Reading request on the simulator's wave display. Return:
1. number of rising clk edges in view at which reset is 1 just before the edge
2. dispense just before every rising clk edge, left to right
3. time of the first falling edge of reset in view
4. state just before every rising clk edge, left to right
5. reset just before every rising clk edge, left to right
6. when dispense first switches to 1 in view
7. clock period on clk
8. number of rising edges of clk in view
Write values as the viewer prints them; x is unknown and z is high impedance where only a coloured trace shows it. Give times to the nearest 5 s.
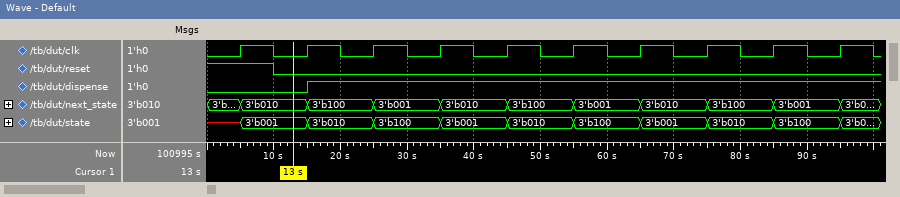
1
0 0 1 1 1 1 1 1 1 1
10 s
x, 3'b001, 3'b010, 3'b100, 3'b001, 3'b010, 3'b100, 3'b001, 3'b010, 3'b100
1 0 0 0 0 0 0 0 0 0
15 s
10 s
10
